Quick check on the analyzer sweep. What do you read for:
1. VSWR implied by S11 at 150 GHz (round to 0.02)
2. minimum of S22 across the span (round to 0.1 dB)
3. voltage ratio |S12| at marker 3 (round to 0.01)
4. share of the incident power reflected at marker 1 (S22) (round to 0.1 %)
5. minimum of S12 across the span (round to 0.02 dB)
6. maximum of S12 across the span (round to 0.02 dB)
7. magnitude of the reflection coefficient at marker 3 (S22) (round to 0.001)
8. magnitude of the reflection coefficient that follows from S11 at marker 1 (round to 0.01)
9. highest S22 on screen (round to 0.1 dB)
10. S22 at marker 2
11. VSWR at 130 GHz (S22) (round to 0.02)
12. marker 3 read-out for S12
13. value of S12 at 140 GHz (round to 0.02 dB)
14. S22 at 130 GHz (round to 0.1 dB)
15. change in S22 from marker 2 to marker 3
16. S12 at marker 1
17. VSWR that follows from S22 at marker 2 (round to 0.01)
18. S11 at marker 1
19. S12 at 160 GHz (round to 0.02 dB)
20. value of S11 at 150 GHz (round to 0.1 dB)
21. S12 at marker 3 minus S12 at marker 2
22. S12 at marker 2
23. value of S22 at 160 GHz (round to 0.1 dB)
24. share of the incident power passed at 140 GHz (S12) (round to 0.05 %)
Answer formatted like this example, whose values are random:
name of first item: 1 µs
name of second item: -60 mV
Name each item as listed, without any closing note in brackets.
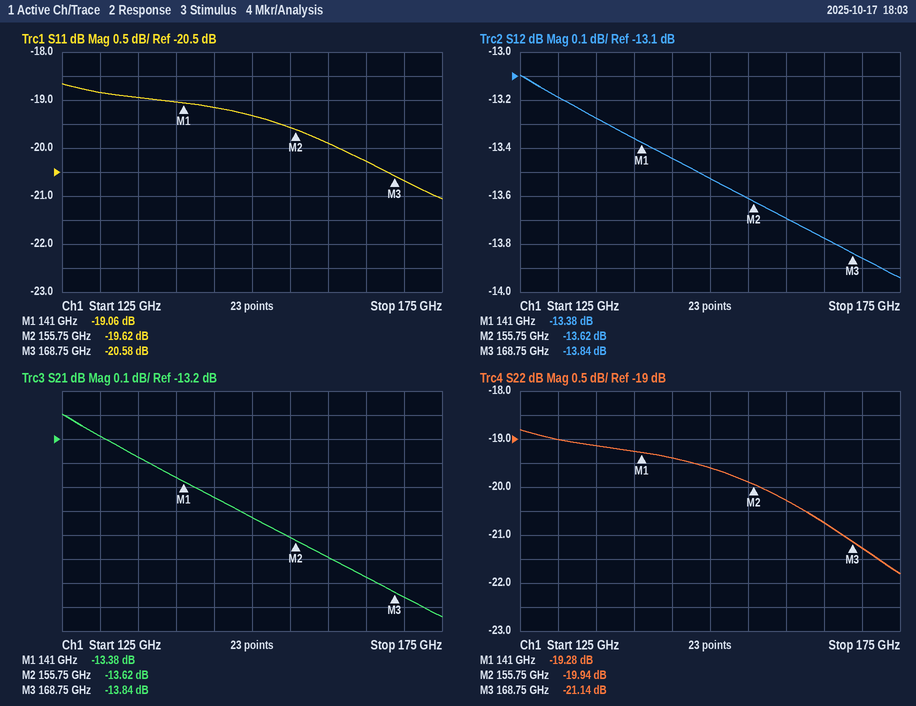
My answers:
VSWR implied by S11 at 150 GHz: 1.24
minimum of S22 across the span: -21.8 dB
voltage ratio |S12| at marker 3: 0.20
share of the incident power reflected at marker 1 (S22): 1.2 %
minimum of S12 across the span: -13.94 dB
maximum of S12 across the span: -13.10 dB
magnitude of the reflection coefficient at marker 3 (S22): 0.088
magnitude of the reflection coefficient that follows from S11 at marker 1: 0.11
highest S22 on screen: -18.8 dB
S22 at marker 2: -19.94 dB
VSWR at 130 GHz (S22): 1.26
marker 3 read-out for S12: -13.84 dB
value of S12 at 140 GHz: -13.36 dB
S22 at 130 GHz: -19.0 dB
change in S22 from marker 2 to marker 3: -1.20 dB
S12 at marker 1: -13.38 dB
VSWR that follows from S22 at marker 2: 1.22
S11 at marker 1: -19.06 dB
S12 at 160 GHz: -13.70 dB
value of S11 at 150 GHz: -19.3 dB
S12 at marker 3 minus S12 at marker 2: -0.22 dB
S12 at marker 2: -13.62 dB
value of S22 at 160 GHz: -20.3 dB
share of the incident power passed at 140 GHz (S12): 4.60 %
